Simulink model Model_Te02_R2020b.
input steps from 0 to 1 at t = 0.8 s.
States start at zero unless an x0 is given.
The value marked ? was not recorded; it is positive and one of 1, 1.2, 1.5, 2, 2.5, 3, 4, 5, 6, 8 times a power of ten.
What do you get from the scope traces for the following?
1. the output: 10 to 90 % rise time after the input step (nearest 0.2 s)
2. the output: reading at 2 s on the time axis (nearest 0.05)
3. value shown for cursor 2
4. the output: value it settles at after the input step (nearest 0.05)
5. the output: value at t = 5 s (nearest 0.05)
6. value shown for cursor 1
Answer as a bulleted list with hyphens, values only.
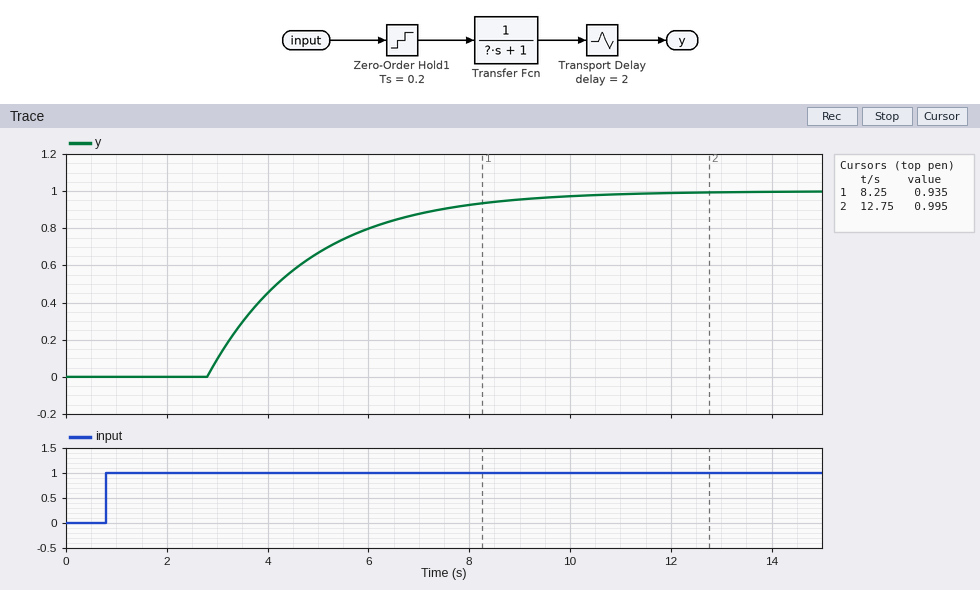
- 4.4 s
- 0.00
- 0.995
- 1.00
- 0.65
- 0.935
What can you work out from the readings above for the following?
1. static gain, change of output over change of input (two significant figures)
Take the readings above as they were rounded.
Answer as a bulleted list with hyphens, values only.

- 1.0
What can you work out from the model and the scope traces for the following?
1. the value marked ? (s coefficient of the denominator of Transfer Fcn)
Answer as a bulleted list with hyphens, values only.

- 2
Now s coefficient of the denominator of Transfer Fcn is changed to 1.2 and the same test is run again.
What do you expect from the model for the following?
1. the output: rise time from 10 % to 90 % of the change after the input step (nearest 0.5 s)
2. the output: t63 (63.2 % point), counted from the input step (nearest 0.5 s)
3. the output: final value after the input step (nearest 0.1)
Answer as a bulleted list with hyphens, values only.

- 2.5 s
- 3.0 s
- 1.0
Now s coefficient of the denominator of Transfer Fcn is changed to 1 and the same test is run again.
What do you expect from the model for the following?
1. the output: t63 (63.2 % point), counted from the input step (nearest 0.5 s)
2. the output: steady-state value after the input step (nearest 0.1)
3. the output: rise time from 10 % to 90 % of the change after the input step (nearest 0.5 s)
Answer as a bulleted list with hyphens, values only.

- 3.0 s
- 1.0
- 2.0 s
